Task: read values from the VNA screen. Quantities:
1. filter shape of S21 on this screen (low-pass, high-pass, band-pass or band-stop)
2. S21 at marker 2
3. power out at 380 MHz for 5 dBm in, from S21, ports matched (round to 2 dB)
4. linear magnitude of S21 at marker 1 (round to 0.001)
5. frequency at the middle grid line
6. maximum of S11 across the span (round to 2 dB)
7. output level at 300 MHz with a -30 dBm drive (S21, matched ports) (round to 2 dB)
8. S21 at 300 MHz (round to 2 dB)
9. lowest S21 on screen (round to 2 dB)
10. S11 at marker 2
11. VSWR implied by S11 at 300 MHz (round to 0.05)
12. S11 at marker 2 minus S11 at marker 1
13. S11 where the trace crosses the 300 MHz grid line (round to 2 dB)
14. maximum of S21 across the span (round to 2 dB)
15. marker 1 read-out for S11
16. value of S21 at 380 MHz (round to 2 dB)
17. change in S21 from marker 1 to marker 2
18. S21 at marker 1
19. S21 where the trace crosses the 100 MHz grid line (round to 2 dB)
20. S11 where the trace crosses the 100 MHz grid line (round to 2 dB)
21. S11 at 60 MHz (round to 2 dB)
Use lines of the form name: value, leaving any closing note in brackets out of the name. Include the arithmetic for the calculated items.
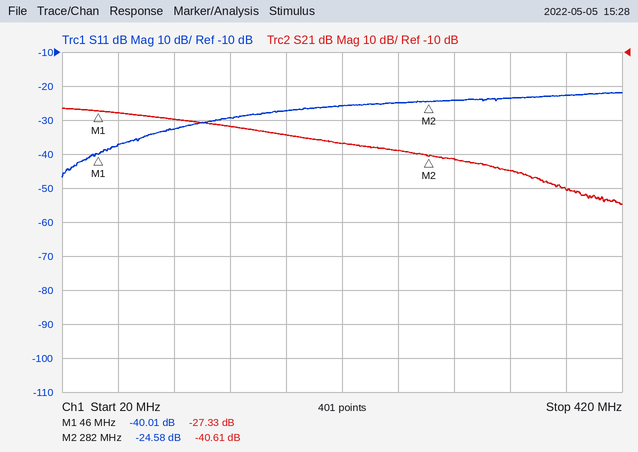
filter shape of S21 on this screen: low-pass
S21 at marker 2: -40.61 dB
power out at 380 MHz for 5 dBm in, from S21, ports matched: 5 dBm + (-50 dB) = -46 dBm
linear magnitude of S21 at marker 1: 10^(-27.33/20) ≈ 0.043
frequency at the middle grid line: 220 MHz
maximum of S11 across the span: -22 dB
output level at 300 MHz with a -30 dBm drive (S21, matched ports): -30 dBm + (-42 dB) = -72 dBm
S21 at 300 MHz: -42 dB
lowest S21 on screen: -54 dB
S11 at marker 2: -24.58 dB
VSWR implied by S11 at 300 MHz: |Γ| = 10^(-24/20) = 0.0631; VSWR = (1 + 0.0631)/(1 − 0.0631) ≈ 1.13, so 1.15 to the nearest 0.05
S11 at marker 2 minus S11 at marker 1: -24.58 − (-40.01) = 15.43 dB
S11 where the trace crosses the 300 MHz grid line: -24 dB
maximum of S21 across the span: -26 dB
marker 1 read-out for S11: -40.01 dB
value of S21 at 380 MHz: -50 dB
change in S21 from marker 1 to marker 2: -40.61 − (-27.33) = -13.28 dB
S21 at marker 1: -27.33 dB
S21 where the trace crosses the 100 MHz grid line: -30 dB
S11 where the trace crosses the 100 MHz grid line: -32 dB
S11 at 60 MHz: -38 dB
